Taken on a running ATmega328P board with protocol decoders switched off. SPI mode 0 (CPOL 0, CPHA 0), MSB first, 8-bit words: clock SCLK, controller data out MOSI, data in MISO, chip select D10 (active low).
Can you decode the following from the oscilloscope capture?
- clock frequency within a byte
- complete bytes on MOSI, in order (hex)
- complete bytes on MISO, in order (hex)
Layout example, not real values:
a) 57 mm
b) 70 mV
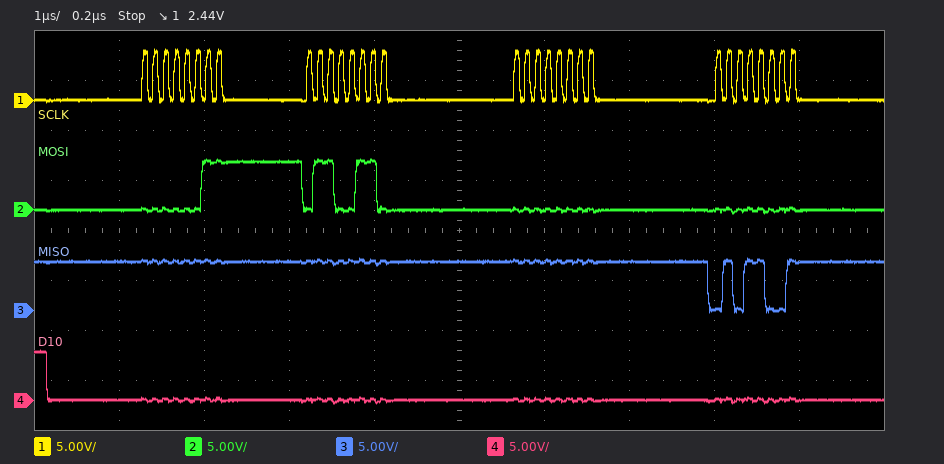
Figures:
a) 8 MHz
b) 03 66 00 00
c) FF FF FF 59
